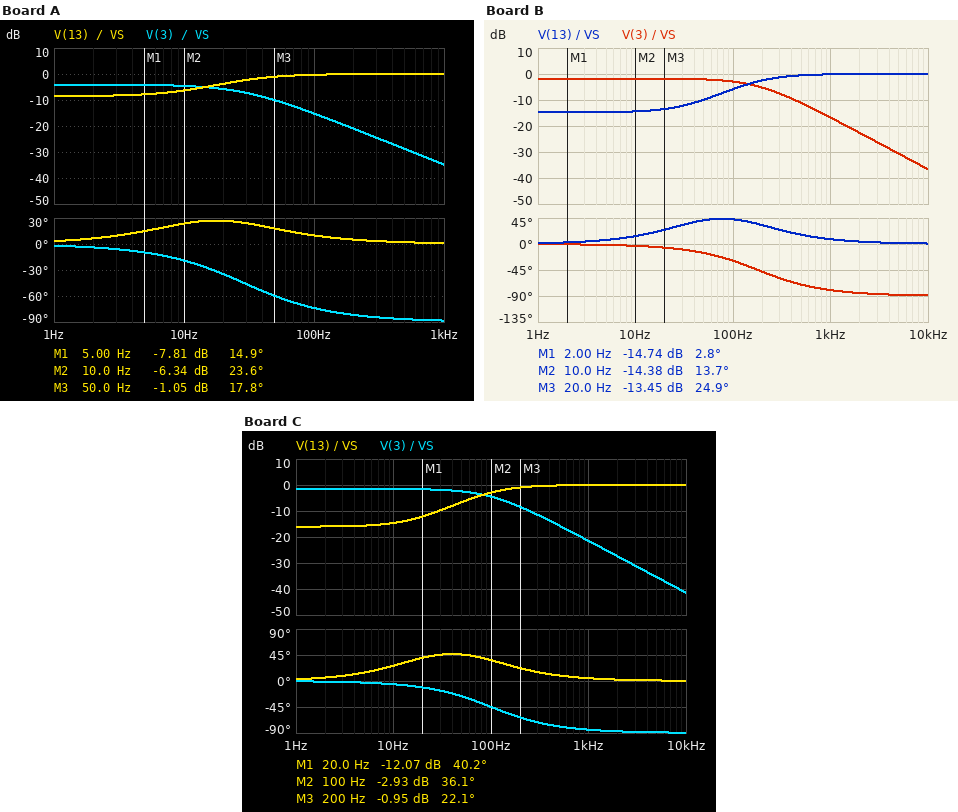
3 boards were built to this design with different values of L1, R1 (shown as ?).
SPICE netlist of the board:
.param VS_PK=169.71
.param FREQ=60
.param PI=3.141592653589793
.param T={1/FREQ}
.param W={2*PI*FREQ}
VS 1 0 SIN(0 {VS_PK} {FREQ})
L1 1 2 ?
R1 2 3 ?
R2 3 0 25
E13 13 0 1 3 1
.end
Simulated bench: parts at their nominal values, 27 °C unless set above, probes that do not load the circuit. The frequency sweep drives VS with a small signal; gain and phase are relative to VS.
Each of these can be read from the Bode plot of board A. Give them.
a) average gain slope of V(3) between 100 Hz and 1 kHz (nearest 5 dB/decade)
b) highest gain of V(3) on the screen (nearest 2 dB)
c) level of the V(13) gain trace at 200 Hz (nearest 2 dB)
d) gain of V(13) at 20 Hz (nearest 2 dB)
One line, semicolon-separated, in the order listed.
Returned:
-20 dB/decade; -4 dB; 0 dB; -4 dB
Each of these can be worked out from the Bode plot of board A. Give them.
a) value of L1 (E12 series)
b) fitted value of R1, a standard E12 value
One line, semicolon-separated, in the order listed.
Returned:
220 mH; 15 Ω
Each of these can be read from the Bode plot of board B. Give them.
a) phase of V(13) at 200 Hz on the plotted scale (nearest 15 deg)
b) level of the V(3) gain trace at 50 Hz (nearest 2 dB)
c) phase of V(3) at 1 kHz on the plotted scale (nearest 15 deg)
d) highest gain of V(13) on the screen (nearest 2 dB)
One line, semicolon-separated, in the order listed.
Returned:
30 deg; -2 dB; -75 deg; 0 dB
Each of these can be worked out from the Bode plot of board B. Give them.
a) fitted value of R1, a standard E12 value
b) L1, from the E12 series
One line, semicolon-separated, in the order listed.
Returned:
5.6 Ω; 27 mH
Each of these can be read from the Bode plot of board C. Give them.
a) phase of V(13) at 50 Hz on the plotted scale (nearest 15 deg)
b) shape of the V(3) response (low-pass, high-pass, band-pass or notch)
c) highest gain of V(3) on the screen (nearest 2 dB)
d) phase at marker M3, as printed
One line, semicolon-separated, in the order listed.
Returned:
45 deg; low-pass; -2 dB; 22.1 deg
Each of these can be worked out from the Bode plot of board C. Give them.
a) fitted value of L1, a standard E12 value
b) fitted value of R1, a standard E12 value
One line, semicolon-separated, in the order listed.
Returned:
47 mH; 4.7 Ω
